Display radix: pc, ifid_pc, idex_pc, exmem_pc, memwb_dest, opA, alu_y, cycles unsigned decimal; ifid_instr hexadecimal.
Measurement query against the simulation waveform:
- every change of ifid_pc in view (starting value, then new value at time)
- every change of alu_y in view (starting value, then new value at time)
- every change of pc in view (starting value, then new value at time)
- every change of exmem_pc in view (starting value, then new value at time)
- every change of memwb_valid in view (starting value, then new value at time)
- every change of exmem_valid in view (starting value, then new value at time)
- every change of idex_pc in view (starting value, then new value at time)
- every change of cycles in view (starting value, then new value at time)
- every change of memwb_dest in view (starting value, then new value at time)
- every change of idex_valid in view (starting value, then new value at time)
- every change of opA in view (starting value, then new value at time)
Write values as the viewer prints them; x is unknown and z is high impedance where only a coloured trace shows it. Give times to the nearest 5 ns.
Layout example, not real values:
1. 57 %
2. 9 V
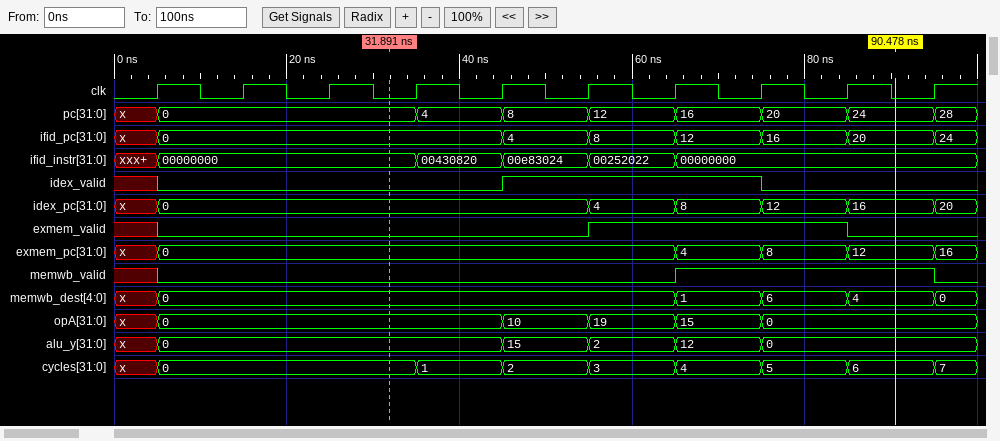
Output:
1. x, 0 at 5 ns, 4 at 45 ns, 8 at 55 ns, 12 at 65 ns, 16 at 75 ns, 20 at 85 ns, 24 at 95 ns
2. x, 0 at 5 ns, 15 at 45 ns, 2 at 55 ns, 12 at 65 ns, 0 at 75 ns
3. x, 0 at 5 ns, 4 at 35 ns, 8 at 45 ns, 12 at 55 ns, 16 at 65 ns, 20 at 75 ns, 24 at 85 ns, 28 at 95 ns
4. x, 0 at 5 ns, 4 at 65 ns, 8 at 75 ns, 12 at 85 ns, 16 at 95 ns
5. x, 0 at 5 ns, 1 at 65 ns, 0 at 95 ns
6. x, 0 at 5 ns, 1 at 55 ns, 0 at 85 ns
7. x, 0 at 5 ns, 4 at 55 ns, 8 at 65 ns, 12 at 75 ns, 16 at 85 ns, 20 at 95 ns
8. x, 0 at 5 ns, 1 at 35 ns, 2 at 45 ns, 3 at 55 ns, 4 at 65 ns, 5 at 75 ns, 6 at 85 ns, 7 at 95 ns
9. x, 0 at 5 ns, 1 at 65 ns, 6 at 75 ns, 4 at 85 ns, 0 at 95 ns
10. x, 0 at 5 ns, 1 at 45 ns, 0 at 75 ns
11. x, 0 at 5 ns, 10 at 45 ns, 19 at 55 ns, 15 at 65 ns, 0 at 75 ns
